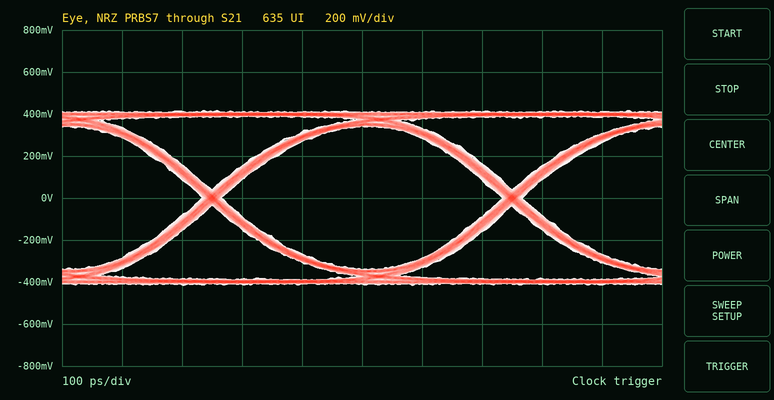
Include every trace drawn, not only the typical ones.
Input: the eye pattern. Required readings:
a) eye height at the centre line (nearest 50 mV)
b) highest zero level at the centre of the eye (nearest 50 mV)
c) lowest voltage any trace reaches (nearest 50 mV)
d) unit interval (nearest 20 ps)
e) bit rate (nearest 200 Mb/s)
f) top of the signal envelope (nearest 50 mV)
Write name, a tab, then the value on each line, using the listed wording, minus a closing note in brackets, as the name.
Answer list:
eye height at the centre line	700 mV
highest zero level at the centre of the eye	-350 mV
lowest voltage any trace reaches	-400 mV
unit interval	500 ps
bit rate	2.0 Gb/s
top of the signal envelope	400 mV
